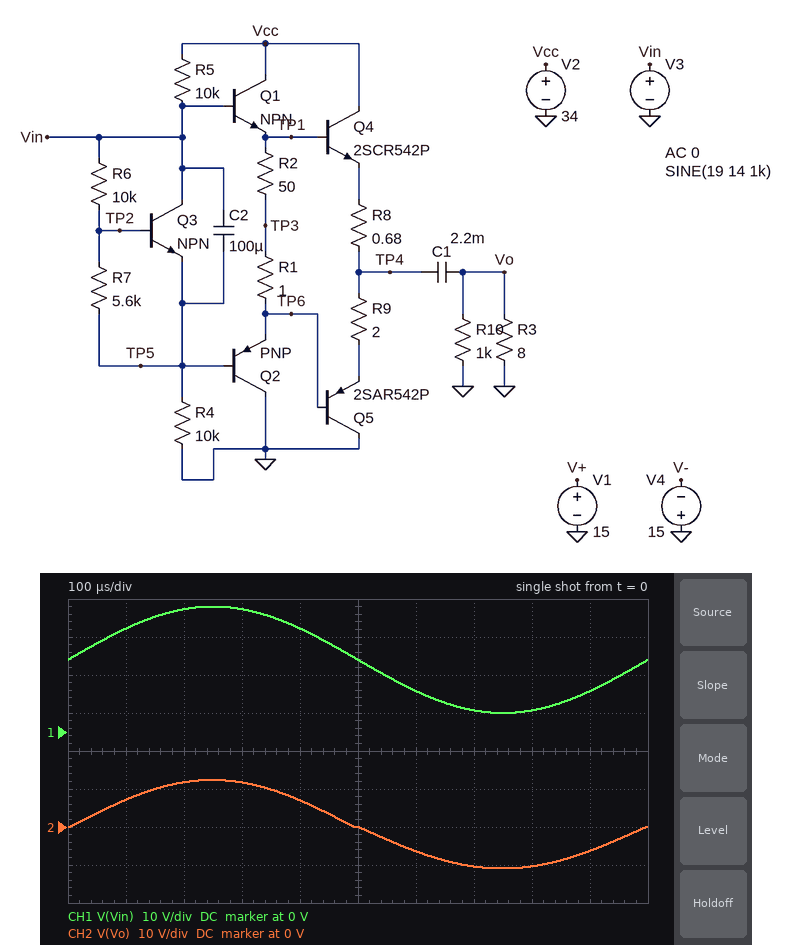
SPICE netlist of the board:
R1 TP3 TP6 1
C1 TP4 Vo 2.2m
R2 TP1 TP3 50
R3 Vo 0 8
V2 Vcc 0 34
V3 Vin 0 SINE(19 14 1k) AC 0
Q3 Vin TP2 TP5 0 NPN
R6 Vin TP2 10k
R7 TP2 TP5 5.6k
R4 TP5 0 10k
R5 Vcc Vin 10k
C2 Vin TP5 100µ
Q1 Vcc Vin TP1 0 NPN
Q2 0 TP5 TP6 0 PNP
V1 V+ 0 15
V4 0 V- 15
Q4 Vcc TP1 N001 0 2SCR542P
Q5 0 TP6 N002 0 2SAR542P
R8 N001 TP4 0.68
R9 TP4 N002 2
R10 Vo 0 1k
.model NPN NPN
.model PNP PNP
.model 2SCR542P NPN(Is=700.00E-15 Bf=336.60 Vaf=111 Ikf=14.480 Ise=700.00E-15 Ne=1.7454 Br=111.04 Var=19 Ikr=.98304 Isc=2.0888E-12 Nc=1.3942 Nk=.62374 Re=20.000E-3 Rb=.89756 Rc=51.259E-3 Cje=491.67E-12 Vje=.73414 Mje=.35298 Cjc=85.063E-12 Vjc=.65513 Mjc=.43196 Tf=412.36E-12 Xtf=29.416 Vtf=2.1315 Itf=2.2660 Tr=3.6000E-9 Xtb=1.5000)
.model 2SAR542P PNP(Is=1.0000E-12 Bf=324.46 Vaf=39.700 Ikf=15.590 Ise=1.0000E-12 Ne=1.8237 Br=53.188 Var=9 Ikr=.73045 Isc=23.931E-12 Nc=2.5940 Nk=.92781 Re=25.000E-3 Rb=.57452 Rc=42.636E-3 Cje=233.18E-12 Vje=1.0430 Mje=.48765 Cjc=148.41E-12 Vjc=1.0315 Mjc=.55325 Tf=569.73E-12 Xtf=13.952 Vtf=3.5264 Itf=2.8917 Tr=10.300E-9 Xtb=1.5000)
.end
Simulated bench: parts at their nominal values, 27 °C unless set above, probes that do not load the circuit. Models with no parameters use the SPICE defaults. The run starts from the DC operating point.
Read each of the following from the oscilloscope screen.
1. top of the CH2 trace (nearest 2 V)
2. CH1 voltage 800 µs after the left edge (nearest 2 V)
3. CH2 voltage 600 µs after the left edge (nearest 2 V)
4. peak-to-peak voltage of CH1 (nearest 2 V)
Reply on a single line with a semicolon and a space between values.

12 V; 6 V; -6 V; 28 V
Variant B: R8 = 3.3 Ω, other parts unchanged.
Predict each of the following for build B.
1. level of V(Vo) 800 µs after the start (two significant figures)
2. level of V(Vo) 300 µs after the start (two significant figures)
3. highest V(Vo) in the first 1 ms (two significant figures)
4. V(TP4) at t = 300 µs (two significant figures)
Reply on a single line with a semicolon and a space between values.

-10 V; 9.0 V; 9.5 V; 27 V
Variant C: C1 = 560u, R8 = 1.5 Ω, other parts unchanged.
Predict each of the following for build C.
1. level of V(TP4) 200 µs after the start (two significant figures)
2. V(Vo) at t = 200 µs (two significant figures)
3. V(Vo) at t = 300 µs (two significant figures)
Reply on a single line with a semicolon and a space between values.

29 V; 11 V; 10 V
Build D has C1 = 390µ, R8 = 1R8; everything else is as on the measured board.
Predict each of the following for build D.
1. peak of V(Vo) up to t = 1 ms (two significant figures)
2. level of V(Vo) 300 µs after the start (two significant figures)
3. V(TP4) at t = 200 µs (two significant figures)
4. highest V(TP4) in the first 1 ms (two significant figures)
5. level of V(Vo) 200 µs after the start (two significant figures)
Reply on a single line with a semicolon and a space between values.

11 V; 9.9 V; 28 V; 29 V; 10 V
